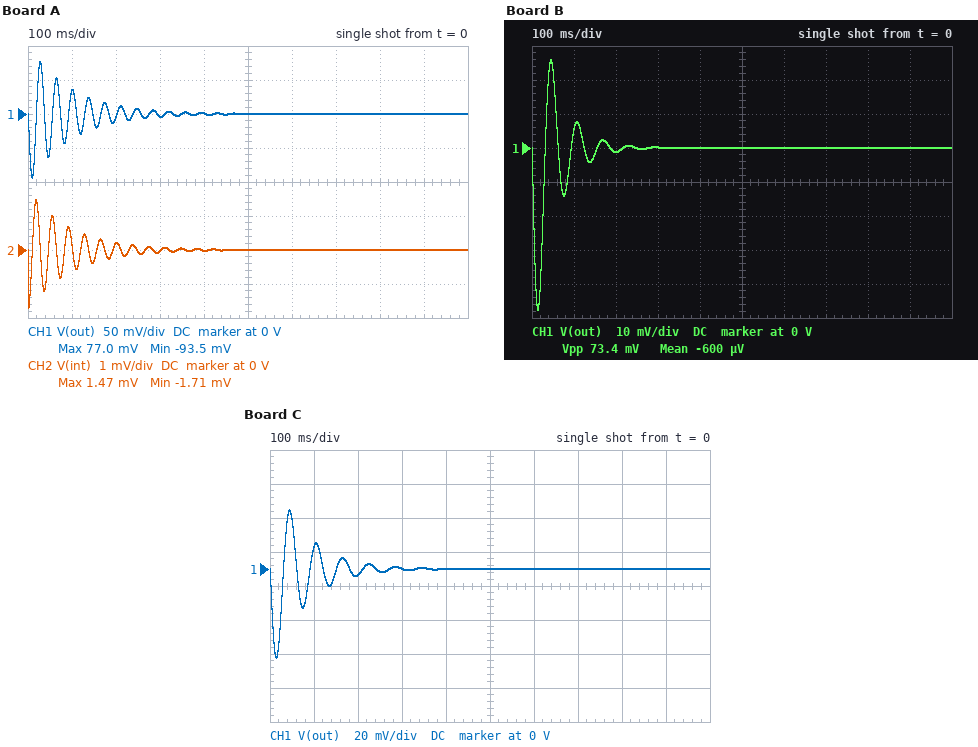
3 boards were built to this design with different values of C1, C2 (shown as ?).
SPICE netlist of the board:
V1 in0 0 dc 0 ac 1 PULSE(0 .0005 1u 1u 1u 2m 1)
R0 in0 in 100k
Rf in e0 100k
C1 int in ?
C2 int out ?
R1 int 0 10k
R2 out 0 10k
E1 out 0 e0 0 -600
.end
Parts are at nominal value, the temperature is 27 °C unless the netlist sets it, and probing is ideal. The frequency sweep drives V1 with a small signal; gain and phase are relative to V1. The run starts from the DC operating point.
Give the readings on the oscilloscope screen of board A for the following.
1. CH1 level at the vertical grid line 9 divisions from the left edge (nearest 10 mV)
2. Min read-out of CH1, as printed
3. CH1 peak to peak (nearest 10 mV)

0 V
-93.5 mV
170 mV
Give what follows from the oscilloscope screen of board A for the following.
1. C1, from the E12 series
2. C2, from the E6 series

5.6 nF
10 nF
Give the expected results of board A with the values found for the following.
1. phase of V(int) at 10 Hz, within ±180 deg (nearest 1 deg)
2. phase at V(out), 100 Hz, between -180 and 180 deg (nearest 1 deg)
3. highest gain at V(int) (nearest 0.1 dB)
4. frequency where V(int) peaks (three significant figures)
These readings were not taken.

-93 deg
8 deg
38.5 dB
27.4 Hz
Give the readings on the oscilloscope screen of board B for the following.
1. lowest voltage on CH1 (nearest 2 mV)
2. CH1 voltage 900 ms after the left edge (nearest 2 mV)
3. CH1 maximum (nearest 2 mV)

-48 mV
0 V
26 mV
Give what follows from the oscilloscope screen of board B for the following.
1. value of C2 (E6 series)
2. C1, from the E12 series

4.7 nF
33 nF
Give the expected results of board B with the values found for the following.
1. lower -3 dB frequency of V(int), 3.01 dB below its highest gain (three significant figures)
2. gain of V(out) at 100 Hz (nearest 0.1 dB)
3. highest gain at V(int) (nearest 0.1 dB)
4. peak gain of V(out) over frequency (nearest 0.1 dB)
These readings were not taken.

13.6 Hz
24.7 dB
17.6 dB
64.1 dB
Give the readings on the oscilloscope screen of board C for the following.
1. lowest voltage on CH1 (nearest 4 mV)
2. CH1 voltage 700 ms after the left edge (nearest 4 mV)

-52 mV
0 V
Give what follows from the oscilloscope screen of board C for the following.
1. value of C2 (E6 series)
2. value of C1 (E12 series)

6.8 nF
22 nF
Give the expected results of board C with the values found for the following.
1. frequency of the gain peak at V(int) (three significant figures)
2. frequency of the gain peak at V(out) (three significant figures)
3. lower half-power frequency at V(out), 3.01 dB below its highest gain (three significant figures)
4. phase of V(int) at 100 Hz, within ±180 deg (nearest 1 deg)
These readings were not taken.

16.8 Hz
16.5 Hz
14.1 Hz
93 deg
